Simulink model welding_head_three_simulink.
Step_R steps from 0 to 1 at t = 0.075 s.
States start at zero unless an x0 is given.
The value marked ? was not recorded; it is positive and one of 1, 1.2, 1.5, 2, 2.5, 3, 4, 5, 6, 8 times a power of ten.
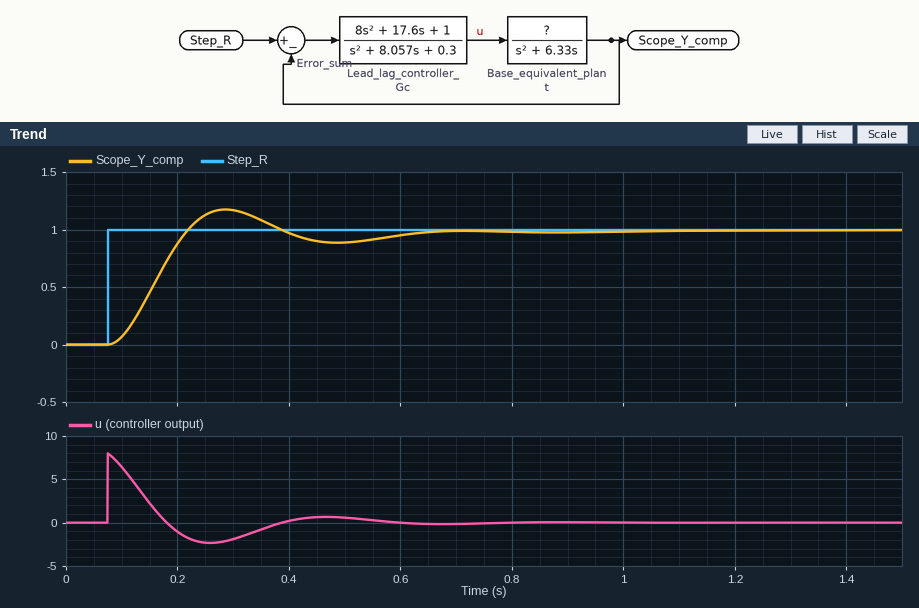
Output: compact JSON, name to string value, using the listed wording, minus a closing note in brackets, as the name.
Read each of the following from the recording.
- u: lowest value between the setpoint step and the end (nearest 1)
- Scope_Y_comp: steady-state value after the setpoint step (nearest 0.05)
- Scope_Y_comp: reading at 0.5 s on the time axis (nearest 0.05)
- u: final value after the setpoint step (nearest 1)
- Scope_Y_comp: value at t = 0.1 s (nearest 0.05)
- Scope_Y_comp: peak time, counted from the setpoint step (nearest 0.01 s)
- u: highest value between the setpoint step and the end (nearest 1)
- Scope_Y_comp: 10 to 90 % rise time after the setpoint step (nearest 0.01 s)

{"u: lowest value between the setpoint step and the end": "-2", "Scope_Y_comp: steady-state value after the setpoint step": "1.00", "Scope_Y_comp: reading at 0.5 s on the time axis": "0.90", "u: final value after the setpoint step": "0", "Scope_Y_comp: value at t = 0.1 s": "0.05", "Scope_Y_comp: peak time, counted from the setpoint step": "0.21 s", "u: highest value between the setpoint step and the end": "8", "Scope_Y_comp: 10 to 90 % rise time after the setpoint step": "0.10 s"}
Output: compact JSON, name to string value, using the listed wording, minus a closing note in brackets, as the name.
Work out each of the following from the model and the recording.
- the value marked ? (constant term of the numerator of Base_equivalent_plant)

{"the value marked ?": "30"}
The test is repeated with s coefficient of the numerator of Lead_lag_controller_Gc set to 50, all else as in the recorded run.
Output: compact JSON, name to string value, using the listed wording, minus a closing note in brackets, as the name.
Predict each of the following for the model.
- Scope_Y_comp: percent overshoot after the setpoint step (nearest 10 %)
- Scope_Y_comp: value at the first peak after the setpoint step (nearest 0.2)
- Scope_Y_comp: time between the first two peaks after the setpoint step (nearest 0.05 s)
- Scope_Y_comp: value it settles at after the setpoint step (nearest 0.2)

{"Scope_Y_comp: percent overshoot after the setpoint step": "40 %", "Scope_Y_comp: value at the first peak after the setpoint step": "1.4", "Scope_Y_comp: time between the first two peaks after the setpoint step": "0.40 s", "Scope_Y_comp: value it settles at after the setpoint step": "1.0"}
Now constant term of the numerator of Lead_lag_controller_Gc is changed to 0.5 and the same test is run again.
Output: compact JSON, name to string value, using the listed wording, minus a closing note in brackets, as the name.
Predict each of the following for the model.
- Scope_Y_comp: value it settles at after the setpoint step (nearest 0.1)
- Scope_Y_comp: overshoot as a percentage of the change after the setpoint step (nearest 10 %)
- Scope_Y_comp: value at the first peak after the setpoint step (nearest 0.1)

{"Scope_Y_comp: value it settles at after the setpoint step": "1.0", "Scope_Y_comp: overshoot as a percentage of the change after the setpoint step": "20 %", "Scope_Y_comp: value at the first peak after the setpoint step": "1.2"}
